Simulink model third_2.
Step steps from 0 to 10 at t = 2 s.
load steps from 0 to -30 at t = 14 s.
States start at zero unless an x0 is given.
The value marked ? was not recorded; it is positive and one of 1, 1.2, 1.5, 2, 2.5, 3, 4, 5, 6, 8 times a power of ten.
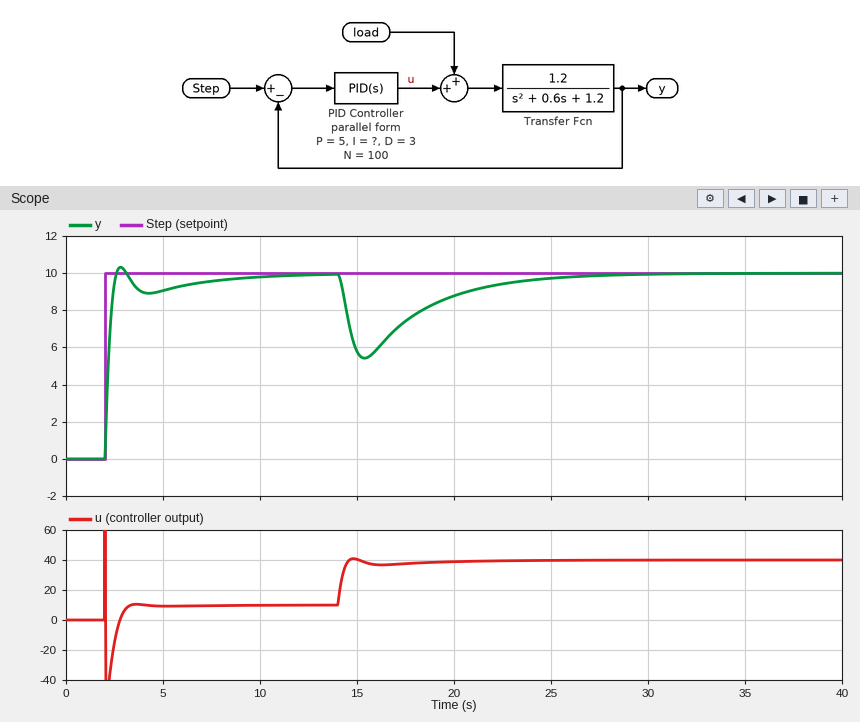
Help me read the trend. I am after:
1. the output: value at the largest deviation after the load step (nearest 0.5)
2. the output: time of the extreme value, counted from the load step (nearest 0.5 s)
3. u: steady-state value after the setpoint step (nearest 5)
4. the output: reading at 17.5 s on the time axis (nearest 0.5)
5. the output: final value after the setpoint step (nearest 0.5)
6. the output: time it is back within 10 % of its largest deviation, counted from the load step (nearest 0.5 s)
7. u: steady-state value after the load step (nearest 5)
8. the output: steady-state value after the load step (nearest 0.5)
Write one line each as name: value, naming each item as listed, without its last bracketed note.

the output: value at the largest deviation after the load step: 5.5
the output: time of the extreme value, counted from the load step: 1.5 s
u: steady-state value after the setpoint step: 10
the output: reading at 17.5 s on the time axis: 7.5
the output: final value after the setpoint step: 10.0
the output: time it is back within 10 % of its largest deviation, counted from the load step: 9.5 s
u: steady-state value after the load step: 40
the output: steady-state value after the load step: 10.0
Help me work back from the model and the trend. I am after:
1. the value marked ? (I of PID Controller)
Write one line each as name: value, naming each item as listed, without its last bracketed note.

the value marked ?: 1.5
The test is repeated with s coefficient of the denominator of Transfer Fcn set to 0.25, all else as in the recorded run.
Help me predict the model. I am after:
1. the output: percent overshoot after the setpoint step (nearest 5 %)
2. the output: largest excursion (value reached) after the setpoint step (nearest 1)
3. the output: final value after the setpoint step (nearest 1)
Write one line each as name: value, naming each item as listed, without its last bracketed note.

the output: percent overshoot after the setpoint step: 10 %
the output: largest excursion (value reached) after the setpoint step: 11
the output: final value after the setpoint step: 10
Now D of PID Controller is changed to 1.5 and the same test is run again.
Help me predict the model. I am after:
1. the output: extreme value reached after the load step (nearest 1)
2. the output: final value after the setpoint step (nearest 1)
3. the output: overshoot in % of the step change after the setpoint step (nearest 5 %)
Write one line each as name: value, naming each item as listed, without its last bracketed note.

the output: extreme value reached after the load step: 4
the output: final value after the setpoint step: 10
the output: overshoot in % of the step change after the setpoint step: 15 %
